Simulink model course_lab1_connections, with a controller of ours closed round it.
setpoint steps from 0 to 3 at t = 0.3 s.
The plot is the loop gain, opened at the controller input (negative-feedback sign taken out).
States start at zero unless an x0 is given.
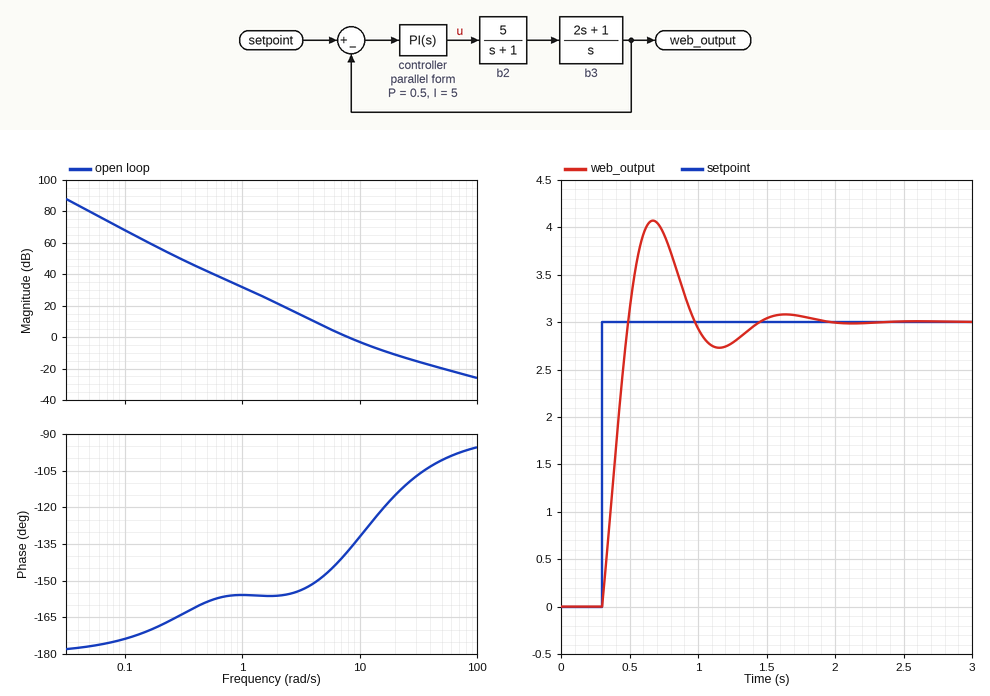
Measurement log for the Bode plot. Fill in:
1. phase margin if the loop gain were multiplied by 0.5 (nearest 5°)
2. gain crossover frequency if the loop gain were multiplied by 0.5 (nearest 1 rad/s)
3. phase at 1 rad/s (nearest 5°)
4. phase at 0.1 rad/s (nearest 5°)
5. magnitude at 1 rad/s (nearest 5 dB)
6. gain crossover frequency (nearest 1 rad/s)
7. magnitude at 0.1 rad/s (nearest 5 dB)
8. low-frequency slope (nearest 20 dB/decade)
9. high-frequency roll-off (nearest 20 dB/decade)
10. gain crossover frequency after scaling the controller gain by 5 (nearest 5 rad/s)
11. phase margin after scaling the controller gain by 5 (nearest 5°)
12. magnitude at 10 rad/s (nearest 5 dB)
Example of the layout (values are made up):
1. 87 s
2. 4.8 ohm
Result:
1. 35°
2. 5 rad/s
3. -155°
4. -175°
5. 30 dB
6. 8 rad/s
7. 70 dB
8. -40 dB/decade
9. -20 dB/decade
10. 25 rad/s
11. 70°
12. -5 dB
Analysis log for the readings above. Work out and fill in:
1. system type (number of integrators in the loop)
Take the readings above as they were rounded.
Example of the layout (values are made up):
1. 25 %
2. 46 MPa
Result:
1. 2
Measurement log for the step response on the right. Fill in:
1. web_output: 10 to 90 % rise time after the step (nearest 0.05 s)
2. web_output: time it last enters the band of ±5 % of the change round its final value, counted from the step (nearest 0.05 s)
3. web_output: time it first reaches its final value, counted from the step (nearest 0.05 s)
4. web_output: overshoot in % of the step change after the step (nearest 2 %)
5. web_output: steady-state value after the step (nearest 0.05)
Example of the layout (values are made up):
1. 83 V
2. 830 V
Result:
1. 0.15 s
2. 1.00 s
3. 0.20 s
4. 36 %
5. 3.00
